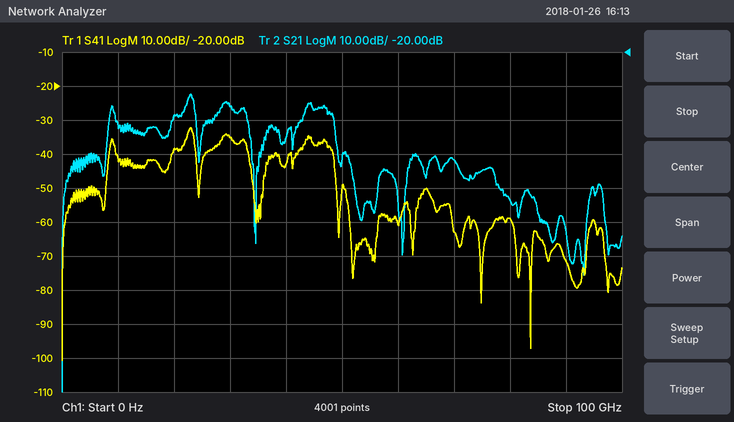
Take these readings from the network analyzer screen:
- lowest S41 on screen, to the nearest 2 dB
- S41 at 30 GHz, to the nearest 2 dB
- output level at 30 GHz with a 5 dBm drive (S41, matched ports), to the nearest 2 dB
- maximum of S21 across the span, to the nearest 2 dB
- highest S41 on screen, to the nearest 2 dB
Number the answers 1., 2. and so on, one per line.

1. -100 dB
2. -36 dB
3. -30 dBm
4. -32 dB
5. -32 dB
